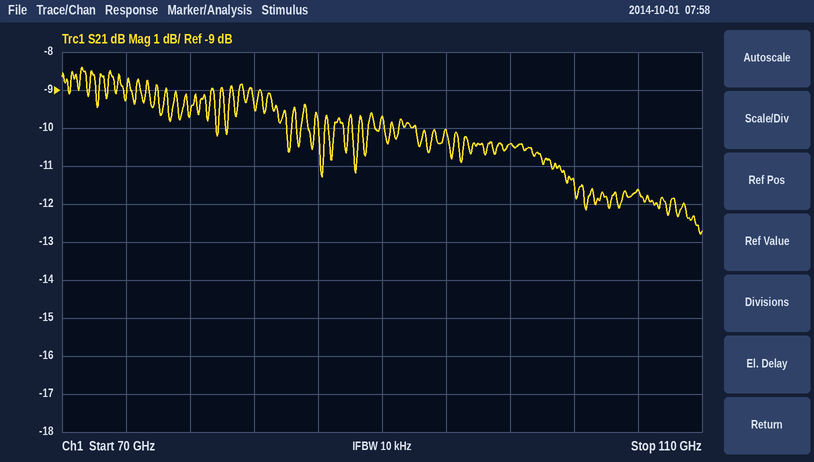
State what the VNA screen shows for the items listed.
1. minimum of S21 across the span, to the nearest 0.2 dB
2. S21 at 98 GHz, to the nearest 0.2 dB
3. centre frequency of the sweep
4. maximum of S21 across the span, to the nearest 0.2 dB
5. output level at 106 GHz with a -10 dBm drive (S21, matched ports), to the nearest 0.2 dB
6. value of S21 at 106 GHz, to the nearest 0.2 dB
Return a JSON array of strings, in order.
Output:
["-12.8 dB", "-10.4 dB", "90 GHz", "-8.4 dB", "-21.6 dBm", "-11.6 dB"]
